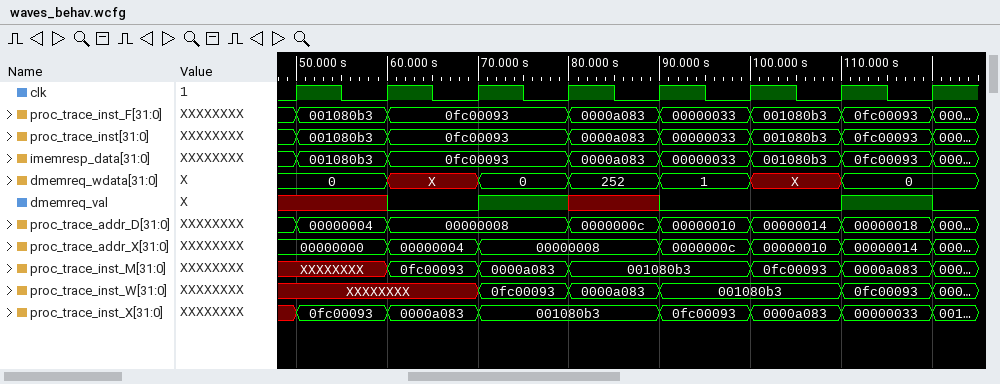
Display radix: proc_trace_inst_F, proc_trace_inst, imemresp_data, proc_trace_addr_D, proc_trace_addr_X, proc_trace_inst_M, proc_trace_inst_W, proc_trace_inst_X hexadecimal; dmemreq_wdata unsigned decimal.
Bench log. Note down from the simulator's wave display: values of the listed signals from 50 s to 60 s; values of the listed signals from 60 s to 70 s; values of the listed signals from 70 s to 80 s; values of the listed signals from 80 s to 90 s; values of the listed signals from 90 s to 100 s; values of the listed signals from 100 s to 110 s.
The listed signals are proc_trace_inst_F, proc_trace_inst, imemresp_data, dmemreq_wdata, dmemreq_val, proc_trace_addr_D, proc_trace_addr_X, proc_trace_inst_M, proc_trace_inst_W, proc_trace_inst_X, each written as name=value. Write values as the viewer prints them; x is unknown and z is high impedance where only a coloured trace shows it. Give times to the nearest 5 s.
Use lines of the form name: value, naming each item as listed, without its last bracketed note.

values of the listed signals from 50 s to 60 s: proc_trace_inst_F=001080b3, proc_trace_inst=001080b3, imemresp_data=001080b3, dmemreq_wdata=0, dmemreq_val=x, proc_trace_addr_D=00000004, proc_trace_addr_X=00000000, proc_trace_inst_M=XXXXXXXX, proc_trace_inst_W=XXXXXXXX, proc_trace_inst_X=0fc00093
values of the listed signals from 60 s to 70 s: proc_trace_inst_F=0fc00093, proc_trace_inst=0fc00093, imemresp_data=0fc00093, dmemreq_wdata=X, dmemreq_val=0, proc_trace_addr_D=00000008, proc_trace_addr_X=00000004, proc_trace_inst_M=0fc00093, proc_trace_inst_W=XXXXXXXX, proc_trace_inst_X=0000a083
values of the listed signals from 70 s to 80 s: proc_trace_inst_F=0fc00093, proc_trace_inst=0fc00093, imemresp_data=0fc00093, dmemreq_wdata=0, dmemreq_val=1, proc_trace_addr_D=00000008, proc_trace_addr_X=00000008, proc_trace_inst_M=0000a083, proc_trace_inst_W=0fc00093, proc_trace_inst_X=001080b3
values of the listed signals from 80 s to 90 s: proc_trace_inst_F=0000a083, proc_trace_inst=0000a083, imemresp_data=0000a083, dmemreq_wdata=252, dmemreq_val=x, proc_trace_addr_D=0000000c, proc_trace_addr_X=00000008, proc_trace_inst_M=001080b3, proc_trace_inst_W=0000a083, proc_trace_inst_X=001080b3
values of the listed signals from 90 s to 100 s: proc_trace_inst_F=00000033, proc_trace_inst=00000033, imemresp_data=00000033, dmemreq_wdata=1, dmemreq_val=0, proc_trace_addr_D=00000010, proc_trace_addr_X=0000000c, proc_trace_inst_M=001080b3, proc_trace_inst_W=001080b3, proc_trace_inst_X=0fc00093
values of the listed signals from 100 s to 110 s: proc_trace_inst_F=001080b3, proc_trace_inst=001080b3, imemresp_data=001080b3, dmemreq_wdata=X, dmemreq_val=0, proc_trace_addr_D=00000014, proc_trace_addr_X=00000010, proc_trace_inst_M=0fc00093, proc_trace_inst_W=001080b3, proc_trace_inst_X=0000a083
